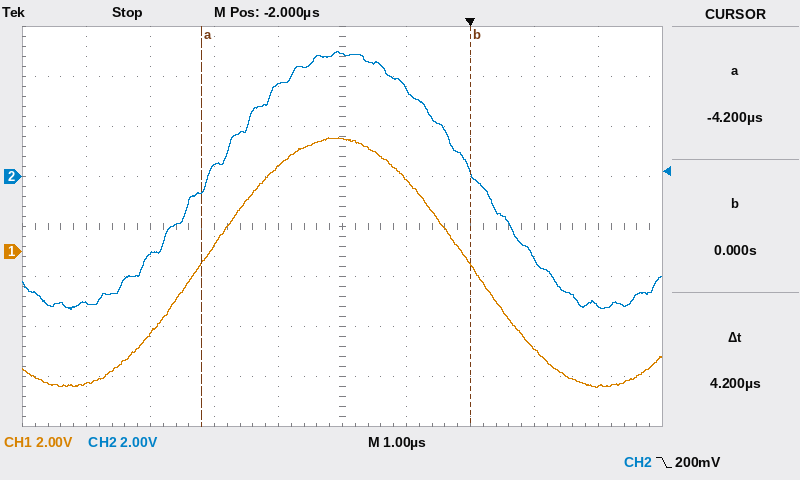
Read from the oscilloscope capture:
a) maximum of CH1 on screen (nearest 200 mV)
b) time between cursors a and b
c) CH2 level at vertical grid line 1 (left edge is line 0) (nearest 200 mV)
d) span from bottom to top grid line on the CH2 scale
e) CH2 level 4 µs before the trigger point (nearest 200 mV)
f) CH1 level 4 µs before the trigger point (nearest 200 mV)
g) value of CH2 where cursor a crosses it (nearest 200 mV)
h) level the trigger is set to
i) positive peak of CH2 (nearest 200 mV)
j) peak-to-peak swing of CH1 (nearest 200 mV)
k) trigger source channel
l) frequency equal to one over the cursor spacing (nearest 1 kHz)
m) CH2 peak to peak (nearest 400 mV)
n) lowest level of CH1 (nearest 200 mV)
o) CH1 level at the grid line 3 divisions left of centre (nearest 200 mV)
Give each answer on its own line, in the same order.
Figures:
4.6 V
4.2 µs
-5.0 V
16 V
400 mV
200 mV
-600 mV
200 mV
5.0 V
10.0 V
CH2
238 kHz
10.4 V
-5.4 V
-3.2 V
